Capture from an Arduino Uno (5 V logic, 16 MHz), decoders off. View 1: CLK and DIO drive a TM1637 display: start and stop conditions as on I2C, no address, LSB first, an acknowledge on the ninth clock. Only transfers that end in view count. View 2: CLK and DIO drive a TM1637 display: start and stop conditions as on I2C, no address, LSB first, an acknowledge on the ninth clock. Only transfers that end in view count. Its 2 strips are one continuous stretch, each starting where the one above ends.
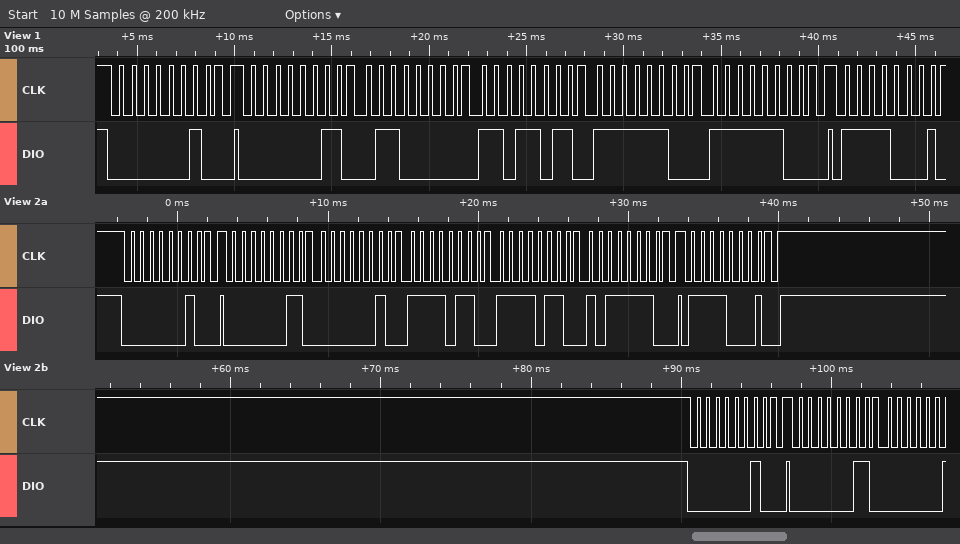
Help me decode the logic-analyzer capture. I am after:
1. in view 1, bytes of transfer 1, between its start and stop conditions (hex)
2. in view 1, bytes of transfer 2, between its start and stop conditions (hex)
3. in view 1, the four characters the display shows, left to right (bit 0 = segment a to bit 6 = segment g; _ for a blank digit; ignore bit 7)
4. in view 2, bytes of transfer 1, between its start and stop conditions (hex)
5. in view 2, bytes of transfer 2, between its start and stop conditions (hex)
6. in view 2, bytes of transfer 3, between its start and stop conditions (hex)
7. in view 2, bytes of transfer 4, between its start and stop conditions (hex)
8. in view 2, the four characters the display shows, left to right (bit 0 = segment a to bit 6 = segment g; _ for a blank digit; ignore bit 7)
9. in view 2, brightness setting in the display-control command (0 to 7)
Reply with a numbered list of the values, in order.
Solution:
1. 40
2. C0 06 DB 3F 3F
3. 1200
4. 40
5. C0 40 6F 6F 7D
6. 8F
7. 40
8. -996
9. 7
